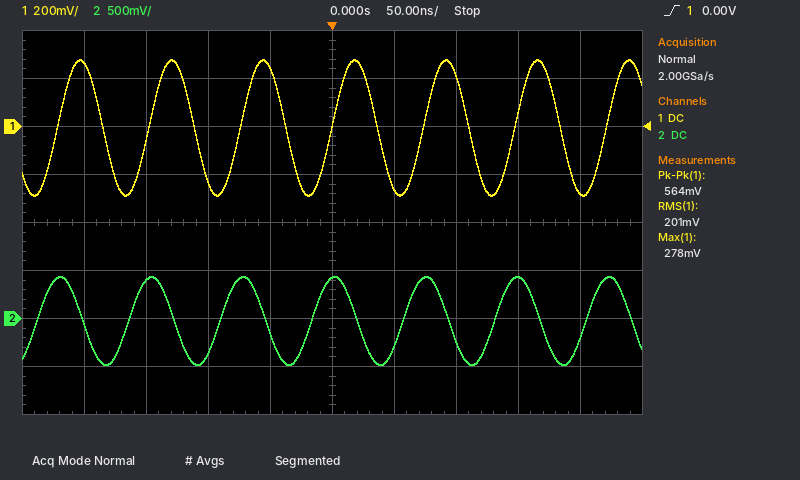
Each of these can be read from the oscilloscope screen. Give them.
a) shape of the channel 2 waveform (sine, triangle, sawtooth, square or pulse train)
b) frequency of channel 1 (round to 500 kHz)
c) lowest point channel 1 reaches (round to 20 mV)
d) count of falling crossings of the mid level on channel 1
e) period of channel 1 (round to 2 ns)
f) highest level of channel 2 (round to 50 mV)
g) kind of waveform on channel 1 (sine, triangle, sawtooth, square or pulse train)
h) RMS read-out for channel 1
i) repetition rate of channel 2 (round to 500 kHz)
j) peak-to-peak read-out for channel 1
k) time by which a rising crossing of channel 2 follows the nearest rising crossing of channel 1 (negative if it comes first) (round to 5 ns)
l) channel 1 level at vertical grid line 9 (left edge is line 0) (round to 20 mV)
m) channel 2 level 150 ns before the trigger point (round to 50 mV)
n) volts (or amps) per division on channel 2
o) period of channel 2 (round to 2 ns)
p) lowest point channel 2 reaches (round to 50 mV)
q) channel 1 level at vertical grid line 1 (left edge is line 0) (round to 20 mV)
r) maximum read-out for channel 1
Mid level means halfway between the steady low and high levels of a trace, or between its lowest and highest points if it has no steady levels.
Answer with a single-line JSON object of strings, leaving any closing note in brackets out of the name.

{"shape of the channel 2 waveform": "sine", "frequency of channel 1": "13.5 MHz", "lowest point channel 1 reaches": "-280 mV", "count of falling crossings of the mid level on channel 1": "6", "period of channel 1": "74 ns", "highest level of channel 2": "450 mV", "kind of waveform on channel 1": "sine", "RMS read-out for channel 1": "201 mV", "repetition rate of channel 2": "13.5 MHz", "peak-to-peak read-out for channel 1": "564 mV", "time by which a rising crossing of channel 2 follows the nearest rising crossing of channel 1 (negative if it comes first)": "-15 ns", "channel 1 level at vertical grid line 9 (left edge is line 0)": "-280 mV", "channel 2 level 150 ns before the trigger point": "400 mV", "volts (or amps) per division on channel 2": "500 mV", "period of channel 2": "74 ns", "lowest point channel 2 reaches": "-500 mV", "channel 1 level at vertical grid line 1 (left edge is line 0)": "260 mV", "maximum read-out for channel 1": "278 mV"}
